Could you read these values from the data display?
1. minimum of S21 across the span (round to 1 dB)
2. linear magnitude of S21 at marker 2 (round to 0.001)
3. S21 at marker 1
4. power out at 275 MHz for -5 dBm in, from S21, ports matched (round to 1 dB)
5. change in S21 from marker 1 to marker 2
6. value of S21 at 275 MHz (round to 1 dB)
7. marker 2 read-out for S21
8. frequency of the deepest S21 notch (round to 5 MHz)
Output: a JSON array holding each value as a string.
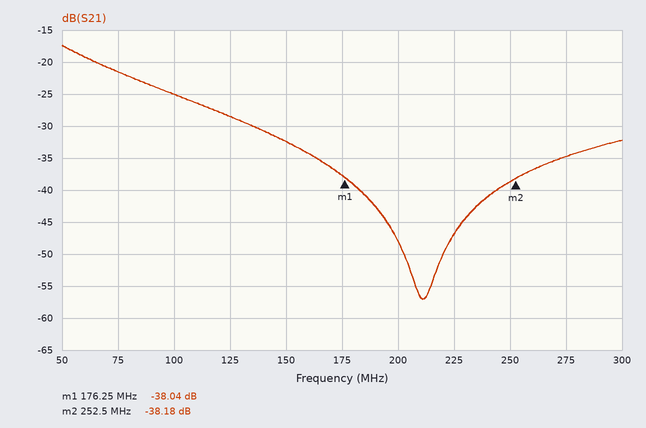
["-57 dB", "0.012", "-38.04 dB", "-40 dBm", "-0.14 dB", "-35 dB", "-38.18 dB", "210 MHz"]
